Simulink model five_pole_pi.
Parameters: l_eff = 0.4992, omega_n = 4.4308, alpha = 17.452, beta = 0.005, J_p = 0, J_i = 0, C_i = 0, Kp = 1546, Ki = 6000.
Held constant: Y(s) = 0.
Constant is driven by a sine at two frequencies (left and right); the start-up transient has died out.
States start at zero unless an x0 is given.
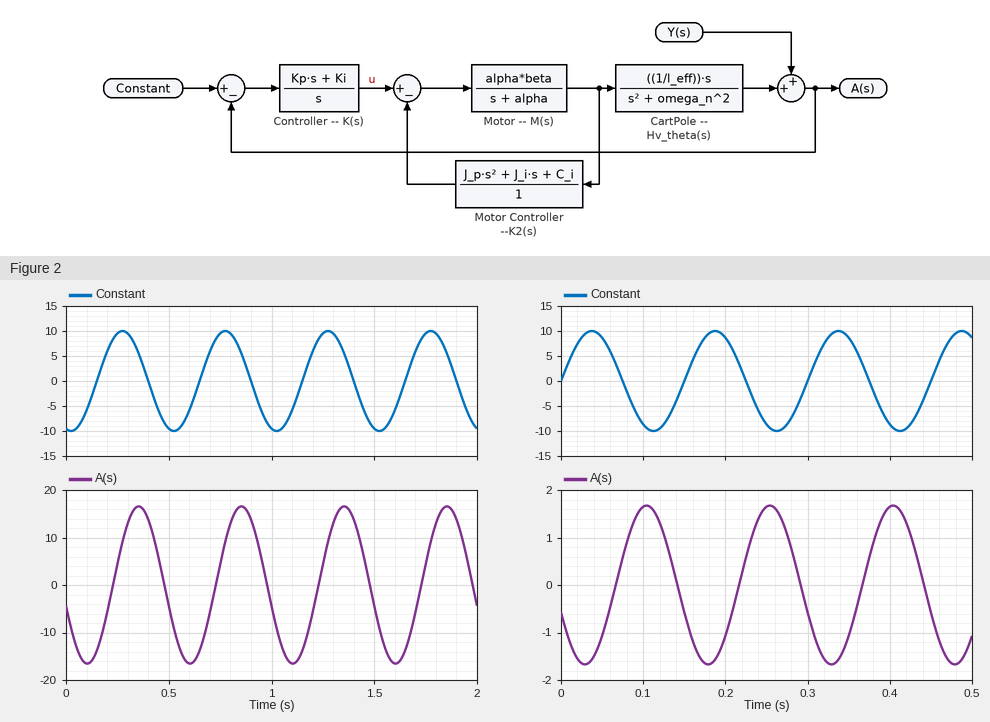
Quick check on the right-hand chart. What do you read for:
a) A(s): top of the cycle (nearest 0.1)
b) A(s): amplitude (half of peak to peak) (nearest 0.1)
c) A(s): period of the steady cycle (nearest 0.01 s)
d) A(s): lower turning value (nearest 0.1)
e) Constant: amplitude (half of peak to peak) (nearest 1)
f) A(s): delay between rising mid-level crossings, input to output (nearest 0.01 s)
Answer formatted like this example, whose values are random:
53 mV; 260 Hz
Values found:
1.7; 1.7; 0.15 s; -1.7; 10; 0.07 s
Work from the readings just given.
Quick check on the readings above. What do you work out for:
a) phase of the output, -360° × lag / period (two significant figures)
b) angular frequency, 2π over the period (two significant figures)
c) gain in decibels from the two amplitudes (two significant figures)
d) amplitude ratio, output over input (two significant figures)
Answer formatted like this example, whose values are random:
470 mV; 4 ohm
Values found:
-170°; 42 rad/s; -15 dB; 0.17
